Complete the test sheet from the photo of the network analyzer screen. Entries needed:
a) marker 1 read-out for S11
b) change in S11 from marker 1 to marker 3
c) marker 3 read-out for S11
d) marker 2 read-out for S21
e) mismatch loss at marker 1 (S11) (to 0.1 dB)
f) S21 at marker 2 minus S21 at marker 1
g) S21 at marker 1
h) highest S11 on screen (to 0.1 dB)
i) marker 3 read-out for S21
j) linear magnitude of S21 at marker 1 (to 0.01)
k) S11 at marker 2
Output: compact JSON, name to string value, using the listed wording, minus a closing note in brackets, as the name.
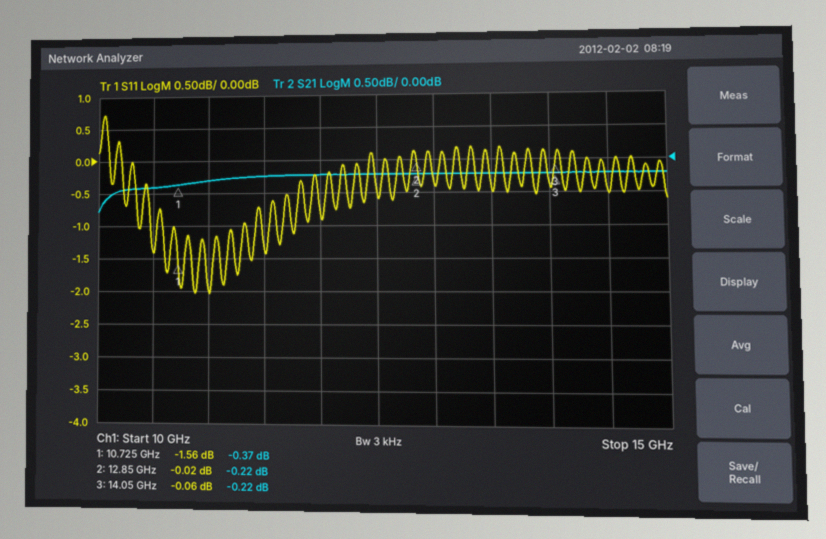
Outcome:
{"marker 1 read-out for S11": "-1.56 dB", "change in S11 from marker 1 to marker 3": "1.50 dB", "marker 3 read-out for S11": "-0.06 dB", "marker 2 read-out for S21": "-0.22 dB", "mismatch loss at marker 1 (S11)": "5.2 dB", "S21 at marker 2 minus S21 at marker 1": "0.15 dB", "S21 at marker 1": "-0.37 dB", "highest S11 on screen": "0.7 dB", "marker 3 read-out for S21": "-0.22 dB", "linear magnitude of S21 at marker 1": "0.96", "S11 at marker 2": "-0.02 dB"}
